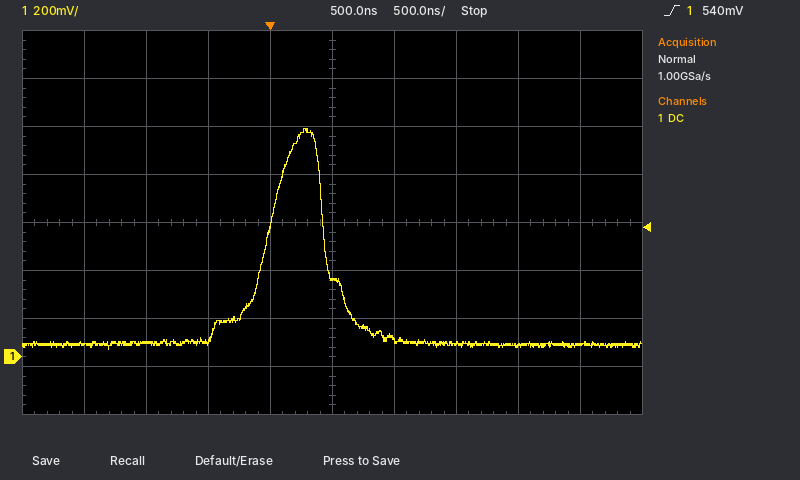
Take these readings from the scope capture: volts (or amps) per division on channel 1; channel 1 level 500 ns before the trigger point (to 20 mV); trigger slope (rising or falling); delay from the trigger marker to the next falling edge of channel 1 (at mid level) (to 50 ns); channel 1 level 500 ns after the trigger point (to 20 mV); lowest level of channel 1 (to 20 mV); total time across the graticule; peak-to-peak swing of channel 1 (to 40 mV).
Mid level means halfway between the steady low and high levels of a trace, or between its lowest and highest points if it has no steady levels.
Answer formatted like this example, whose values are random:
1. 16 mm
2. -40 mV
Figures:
1. 200 mV
2. 60 mV
3. rising
4. 450 ns
5. 340 mV
6. 40 mV
7. 5 µs
8. 920 mV
